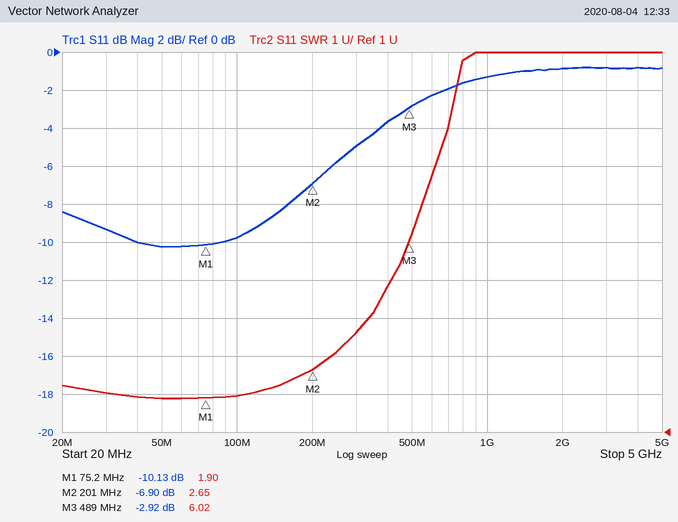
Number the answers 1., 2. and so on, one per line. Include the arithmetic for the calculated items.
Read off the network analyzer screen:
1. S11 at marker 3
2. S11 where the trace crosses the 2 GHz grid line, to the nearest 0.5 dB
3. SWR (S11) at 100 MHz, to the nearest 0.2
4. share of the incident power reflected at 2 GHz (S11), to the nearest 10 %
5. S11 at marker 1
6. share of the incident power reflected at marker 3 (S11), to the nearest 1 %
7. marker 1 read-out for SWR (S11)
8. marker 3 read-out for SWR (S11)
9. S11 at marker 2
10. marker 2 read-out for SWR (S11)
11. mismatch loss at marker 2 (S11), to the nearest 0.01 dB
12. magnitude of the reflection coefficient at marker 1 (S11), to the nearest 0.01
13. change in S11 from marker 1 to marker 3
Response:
1. -2.92 dB
2. -1.0 dB
3. 2.0
4. 10^(-1/10) ≈ 79.4 %, so 80 % to the nearest 10 %
5. -10.13 dB
6. 10^(-2.92/10) ≈ 51 %
7. 1.90
8. 6.02
9. -6.90 dB
10. 2.65
11. −10 log10(1 − 10^(-6.9/10)) ≈ 0.99 dB
12. 10^(-10.13/20) ≈ 0.31
13. -2.92 − (-10.13) = 7.21 dB
